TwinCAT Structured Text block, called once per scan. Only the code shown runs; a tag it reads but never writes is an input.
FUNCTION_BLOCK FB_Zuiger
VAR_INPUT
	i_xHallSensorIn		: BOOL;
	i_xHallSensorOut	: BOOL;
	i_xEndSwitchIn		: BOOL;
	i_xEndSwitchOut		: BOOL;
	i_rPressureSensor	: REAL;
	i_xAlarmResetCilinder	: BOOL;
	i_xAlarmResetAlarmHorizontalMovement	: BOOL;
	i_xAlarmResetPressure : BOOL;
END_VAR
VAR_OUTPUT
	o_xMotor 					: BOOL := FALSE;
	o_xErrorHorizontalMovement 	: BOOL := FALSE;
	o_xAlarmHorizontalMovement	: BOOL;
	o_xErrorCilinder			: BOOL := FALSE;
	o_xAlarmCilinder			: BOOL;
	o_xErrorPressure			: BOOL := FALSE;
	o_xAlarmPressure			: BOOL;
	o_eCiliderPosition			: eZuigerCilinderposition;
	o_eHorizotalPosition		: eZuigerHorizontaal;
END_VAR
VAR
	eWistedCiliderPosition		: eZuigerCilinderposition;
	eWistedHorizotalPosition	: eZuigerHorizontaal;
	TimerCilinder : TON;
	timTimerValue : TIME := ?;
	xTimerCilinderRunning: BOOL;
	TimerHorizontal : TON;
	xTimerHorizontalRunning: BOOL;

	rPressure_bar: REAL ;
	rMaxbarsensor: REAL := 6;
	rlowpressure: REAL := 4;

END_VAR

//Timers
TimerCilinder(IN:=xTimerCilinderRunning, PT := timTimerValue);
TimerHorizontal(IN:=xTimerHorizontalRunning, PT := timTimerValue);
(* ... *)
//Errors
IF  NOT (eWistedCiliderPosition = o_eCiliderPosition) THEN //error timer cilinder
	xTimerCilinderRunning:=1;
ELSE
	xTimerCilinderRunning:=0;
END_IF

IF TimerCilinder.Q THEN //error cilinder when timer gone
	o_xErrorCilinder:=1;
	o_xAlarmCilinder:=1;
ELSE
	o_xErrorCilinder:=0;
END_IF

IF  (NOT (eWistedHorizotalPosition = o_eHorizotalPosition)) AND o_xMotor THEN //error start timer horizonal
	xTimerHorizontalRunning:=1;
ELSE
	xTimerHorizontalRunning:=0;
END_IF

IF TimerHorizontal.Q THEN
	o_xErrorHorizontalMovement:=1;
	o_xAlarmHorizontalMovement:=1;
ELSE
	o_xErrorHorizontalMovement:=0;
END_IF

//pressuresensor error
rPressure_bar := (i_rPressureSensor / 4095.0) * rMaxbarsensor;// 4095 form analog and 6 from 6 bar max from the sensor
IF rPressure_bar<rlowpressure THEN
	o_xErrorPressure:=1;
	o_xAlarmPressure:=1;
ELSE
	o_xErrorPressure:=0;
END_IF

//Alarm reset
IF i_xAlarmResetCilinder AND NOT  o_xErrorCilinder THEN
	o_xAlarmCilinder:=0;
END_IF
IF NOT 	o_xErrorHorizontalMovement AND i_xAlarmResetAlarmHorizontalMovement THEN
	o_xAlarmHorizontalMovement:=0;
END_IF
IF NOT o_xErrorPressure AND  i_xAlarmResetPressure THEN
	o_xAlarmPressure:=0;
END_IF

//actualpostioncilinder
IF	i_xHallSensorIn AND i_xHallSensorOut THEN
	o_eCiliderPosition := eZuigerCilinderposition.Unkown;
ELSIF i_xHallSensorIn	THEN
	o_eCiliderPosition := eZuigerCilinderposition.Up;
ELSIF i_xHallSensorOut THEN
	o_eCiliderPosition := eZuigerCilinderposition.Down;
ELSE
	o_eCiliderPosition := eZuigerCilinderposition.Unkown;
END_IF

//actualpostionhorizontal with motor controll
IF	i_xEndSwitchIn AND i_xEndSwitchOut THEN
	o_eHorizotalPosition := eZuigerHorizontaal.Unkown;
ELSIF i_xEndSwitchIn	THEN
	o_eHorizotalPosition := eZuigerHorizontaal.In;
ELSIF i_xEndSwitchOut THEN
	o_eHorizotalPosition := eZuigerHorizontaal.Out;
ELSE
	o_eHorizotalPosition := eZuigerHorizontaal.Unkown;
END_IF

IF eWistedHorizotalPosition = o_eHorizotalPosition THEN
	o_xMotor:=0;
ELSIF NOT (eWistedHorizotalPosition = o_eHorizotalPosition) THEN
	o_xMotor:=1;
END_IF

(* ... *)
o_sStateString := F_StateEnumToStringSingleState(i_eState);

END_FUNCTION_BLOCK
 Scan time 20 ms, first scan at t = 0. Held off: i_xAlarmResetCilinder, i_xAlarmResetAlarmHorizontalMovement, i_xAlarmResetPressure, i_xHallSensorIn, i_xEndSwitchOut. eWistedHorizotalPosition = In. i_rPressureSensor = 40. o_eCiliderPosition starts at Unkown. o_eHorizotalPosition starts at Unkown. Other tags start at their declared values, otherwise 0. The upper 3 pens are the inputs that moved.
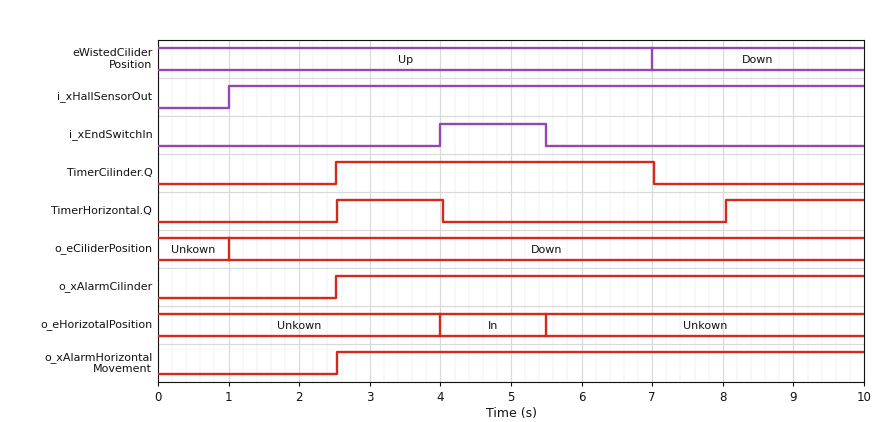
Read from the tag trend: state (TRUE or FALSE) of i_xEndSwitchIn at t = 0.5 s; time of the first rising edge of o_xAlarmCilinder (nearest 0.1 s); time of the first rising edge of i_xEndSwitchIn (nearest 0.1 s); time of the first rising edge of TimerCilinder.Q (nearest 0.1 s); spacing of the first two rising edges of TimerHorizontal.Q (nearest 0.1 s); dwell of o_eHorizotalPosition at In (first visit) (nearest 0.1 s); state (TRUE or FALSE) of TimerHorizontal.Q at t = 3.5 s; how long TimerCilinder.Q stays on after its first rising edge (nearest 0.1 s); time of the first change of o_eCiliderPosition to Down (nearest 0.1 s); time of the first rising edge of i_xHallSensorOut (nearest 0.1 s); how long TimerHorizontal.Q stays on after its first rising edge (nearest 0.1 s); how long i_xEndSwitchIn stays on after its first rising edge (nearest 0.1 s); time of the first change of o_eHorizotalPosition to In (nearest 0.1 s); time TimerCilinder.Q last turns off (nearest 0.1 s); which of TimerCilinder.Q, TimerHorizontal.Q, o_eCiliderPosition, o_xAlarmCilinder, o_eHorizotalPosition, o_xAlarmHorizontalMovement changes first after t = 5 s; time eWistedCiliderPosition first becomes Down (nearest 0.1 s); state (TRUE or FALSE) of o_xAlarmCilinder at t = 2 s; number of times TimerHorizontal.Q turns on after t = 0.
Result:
FALSE
2.5 s
4.0 s
2.5 s
5.5 s
1.5 s
TRUE
4.5 s
1.0 s
1.0 s
1.5 s
1.5 s
4.0 s
7.0 s
o_eHorizotalPosition
7.0 s
FALSE
2
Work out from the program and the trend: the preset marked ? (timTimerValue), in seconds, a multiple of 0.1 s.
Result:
2.5 s
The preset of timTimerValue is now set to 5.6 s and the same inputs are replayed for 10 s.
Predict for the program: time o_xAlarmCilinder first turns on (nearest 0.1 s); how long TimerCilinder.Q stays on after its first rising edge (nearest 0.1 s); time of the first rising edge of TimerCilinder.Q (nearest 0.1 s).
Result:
5.6 s
1.4 s
5.6 s
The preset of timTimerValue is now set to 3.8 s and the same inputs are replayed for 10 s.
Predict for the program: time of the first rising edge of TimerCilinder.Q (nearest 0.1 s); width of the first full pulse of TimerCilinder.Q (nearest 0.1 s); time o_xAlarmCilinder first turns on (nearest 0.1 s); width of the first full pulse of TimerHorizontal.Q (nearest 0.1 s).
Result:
3.8 s
3.2 s
3.8 s
0.2 s
